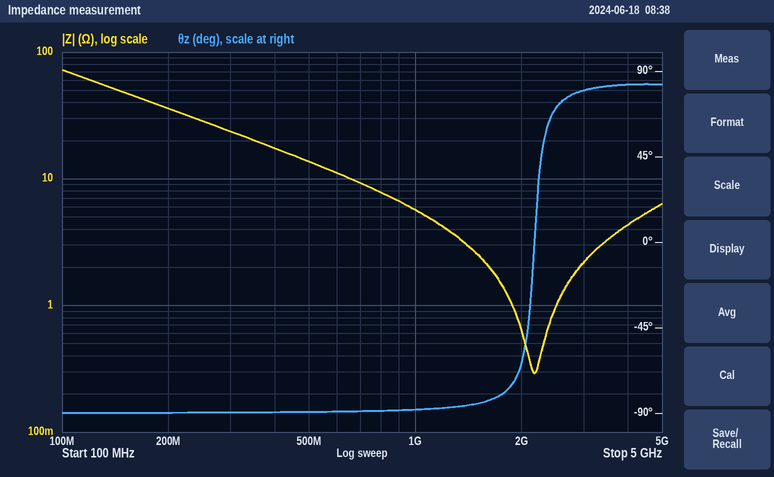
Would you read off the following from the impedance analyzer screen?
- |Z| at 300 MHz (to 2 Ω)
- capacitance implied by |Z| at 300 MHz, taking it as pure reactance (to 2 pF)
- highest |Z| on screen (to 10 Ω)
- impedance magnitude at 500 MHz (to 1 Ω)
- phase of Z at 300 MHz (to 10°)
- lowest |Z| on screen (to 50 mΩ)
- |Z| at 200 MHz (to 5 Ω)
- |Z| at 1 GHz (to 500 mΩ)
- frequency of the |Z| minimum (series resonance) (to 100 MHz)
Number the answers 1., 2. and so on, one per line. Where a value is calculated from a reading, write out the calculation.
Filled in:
1. 24 Ω
2. C = 1/(2π × 300 MHz × 24 Ω) ≈ 22 pF
3. 70 Ω
4. 14 Ω
5. -90°
6. 300 mΩ
7. 35 Ω
8. 5.5 Ω
9. 2.2 GHz
